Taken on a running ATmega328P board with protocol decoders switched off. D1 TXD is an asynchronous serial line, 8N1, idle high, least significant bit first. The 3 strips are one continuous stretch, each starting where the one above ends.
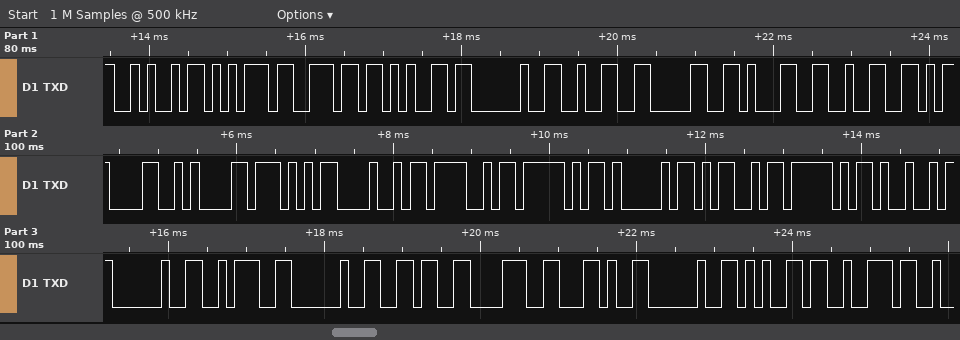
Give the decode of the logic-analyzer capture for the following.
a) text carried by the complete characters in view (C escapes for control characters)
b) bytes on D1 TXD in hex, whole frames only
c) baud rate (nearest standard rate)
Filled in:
"June 2012\r\nWHO_AM_I : 68, er"
4A 75 6E 65 20 32 30 31 32 0D 0A 57 48 4F 5F 41 4D 5F 49 20 3A 20 36 38 2C 20 65 72
9600 baud
